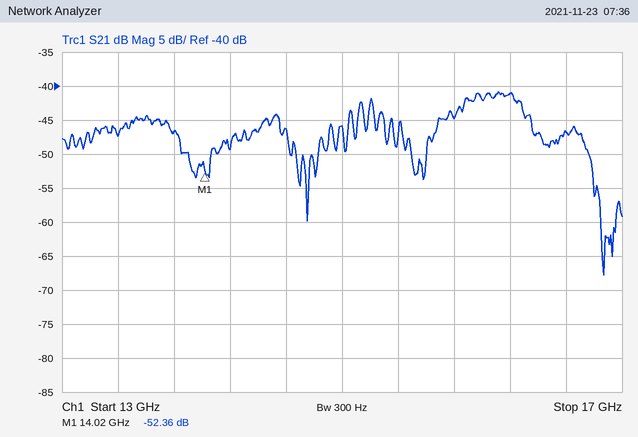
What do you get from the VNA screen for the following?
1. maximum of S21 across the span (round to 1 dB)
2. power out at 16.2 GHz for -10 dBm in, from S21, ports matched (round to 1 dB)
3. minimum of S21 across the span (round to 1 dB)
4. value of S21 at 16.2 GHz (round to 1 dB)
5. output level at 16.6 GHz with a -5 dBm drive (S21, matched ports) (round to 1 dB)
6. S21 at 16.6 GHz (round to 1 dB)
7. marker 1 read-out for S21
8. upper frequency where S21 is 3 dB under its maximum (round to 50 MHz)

-41 dB
-51 dBm
-68 dB
-41 dB
-52 dBm
-47 dB
-52.36 dB
16.30 GHz
